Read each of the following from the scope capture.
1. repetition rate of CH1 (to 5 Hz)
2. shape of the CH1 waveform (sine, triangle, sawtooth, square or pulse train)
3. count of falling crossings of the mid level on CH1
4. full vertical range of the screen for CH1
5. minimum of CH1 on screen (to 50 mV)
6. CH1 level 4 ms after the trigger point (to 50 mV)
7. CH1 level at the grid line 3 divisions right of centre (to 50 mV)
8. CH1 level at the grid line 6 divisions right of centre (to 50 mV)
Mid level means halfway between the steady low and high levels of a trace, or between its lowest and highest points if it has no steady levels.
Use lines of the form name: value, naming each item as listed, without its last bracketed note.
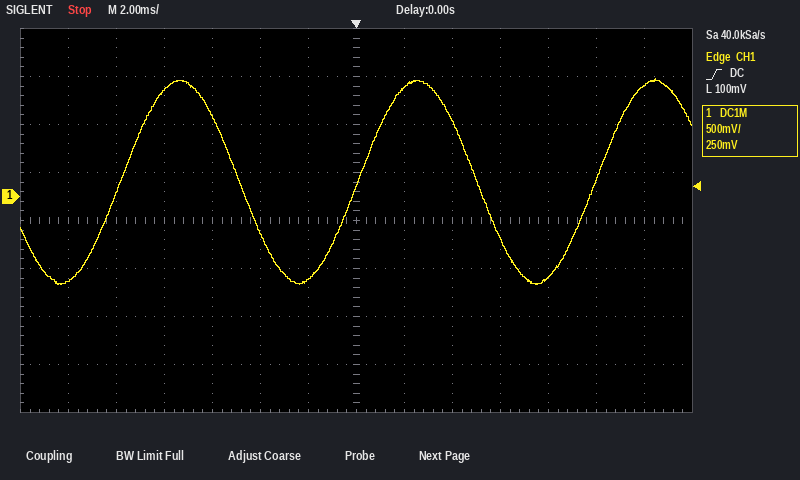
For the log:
repetition rate of CH1: 100 Hz
shape of the CH1 waveform: sine
count of falling crossings of the mid level on CH1: 2
full vertical range of the screen for CH1: 4 V
minimum of CH1 on screen: -900 mV
CH1 level 4 ms after the trigger point: 800 mV
CH1 level at the grid line 3 divisions right of centre: -450 mV
CH1 level at the grid line 6 divisions right of centre: 1.15 V
